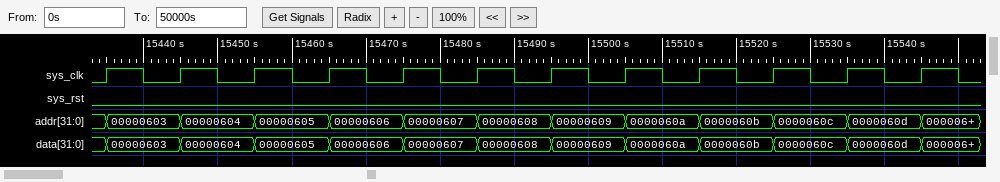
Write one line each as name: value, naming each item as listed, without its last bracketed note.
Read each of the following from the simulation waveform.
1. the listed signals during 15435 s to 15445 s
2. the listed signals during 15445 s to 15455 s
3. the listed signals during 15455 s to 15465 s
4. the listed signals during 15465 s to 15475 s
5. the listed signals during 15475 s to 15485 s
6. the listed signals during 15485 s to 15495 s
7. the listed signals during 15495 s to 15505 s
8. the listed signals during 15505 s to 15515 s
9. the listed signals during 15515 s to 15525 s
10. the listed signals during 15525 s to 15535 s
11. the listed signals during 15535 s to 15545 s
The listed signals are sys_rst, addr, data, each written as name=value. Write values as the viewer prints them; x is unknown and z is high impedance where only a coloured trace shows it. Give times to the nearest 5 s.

the listed signals during 15435 s to 15445 s: sys_rst=0, addr=00000603, data=00000603
the listed signals during 15445 s to 15455 s: sys_rst=0, addr=00000604, data=00000604
the listed signals during 15455 s to 15465 s: sys_rst=0, addr=00000605, data=00000605
the listed signals during 15465 s to 15475 s: sys_rst=0, addr=00000606, data=00000606
the listed signals during 15475 s to 15485 s: sys_rst=0, addr=00000607, data=00000607
the listed signals during 15485 s to 15495 s: sys_rst=0, addr=00000608, data=00000608
the listed signals during 15495 s to 15505 s: sys_rst=0, addr=00000609, data=00000609
the listed signals during 15505 s to 15515 s: sys_rst=0, addr=0000060a, data=0000060a
the listed signals during 15515 s to 15525 s: sys_rst=0, addr=0000060b, data=0000060b
the listed signals during 15525 s to 15535 s: sys_rst=0, addr=0000060c, data=0000060c
the listed signals during 15535 s to 15545 s: sys_rst=0, addr=0000060d, data=0000060d
